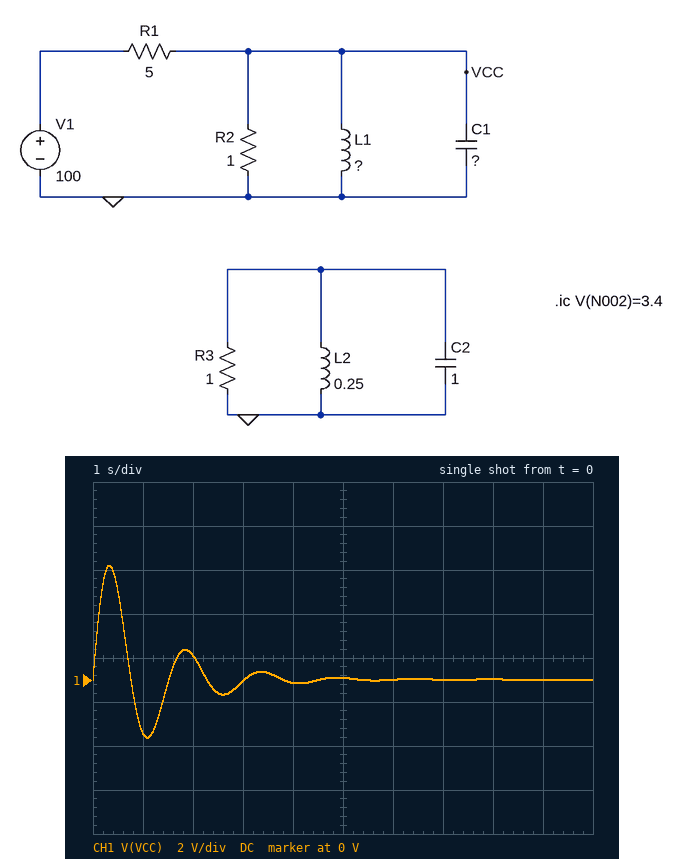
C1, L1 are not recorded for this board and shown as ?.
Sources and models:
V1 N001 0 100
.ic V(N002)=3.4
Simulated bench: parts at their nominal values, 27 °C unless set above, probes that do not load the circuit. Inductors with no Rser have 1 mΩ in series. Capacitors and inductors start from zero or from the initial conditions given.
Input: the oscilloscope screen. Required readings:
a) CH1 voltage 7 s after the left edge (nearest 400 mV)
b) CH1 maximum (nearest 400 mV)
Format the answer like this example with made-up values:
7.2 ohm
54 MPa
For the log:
0 V
5.2 V
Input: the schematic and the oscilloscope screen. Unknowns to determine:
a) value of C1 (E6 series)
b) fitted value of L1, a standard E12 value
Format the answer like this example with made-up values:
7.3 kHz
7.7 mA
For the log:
680 mF
82 mH
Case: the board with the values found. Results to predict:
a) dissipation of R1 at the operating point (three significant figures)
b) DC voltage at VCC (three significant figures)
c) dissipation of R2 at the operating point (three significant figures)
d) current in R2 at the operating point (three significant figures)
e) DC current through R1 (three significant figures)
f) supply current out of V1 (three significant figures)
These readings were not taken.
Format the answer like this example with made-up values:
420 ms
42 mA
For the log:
2.00 kW
20.0 mV
399 µW
20.0 mA
20.0 A
20.0 A
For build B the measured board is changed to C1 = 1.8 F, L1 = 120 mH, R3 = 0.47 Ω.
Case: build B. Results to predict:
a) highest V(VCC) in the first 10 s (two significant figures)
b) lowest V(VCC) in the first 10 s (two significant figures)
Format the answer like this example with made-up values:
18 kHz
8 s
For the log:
4.1 V
-2.5 V
